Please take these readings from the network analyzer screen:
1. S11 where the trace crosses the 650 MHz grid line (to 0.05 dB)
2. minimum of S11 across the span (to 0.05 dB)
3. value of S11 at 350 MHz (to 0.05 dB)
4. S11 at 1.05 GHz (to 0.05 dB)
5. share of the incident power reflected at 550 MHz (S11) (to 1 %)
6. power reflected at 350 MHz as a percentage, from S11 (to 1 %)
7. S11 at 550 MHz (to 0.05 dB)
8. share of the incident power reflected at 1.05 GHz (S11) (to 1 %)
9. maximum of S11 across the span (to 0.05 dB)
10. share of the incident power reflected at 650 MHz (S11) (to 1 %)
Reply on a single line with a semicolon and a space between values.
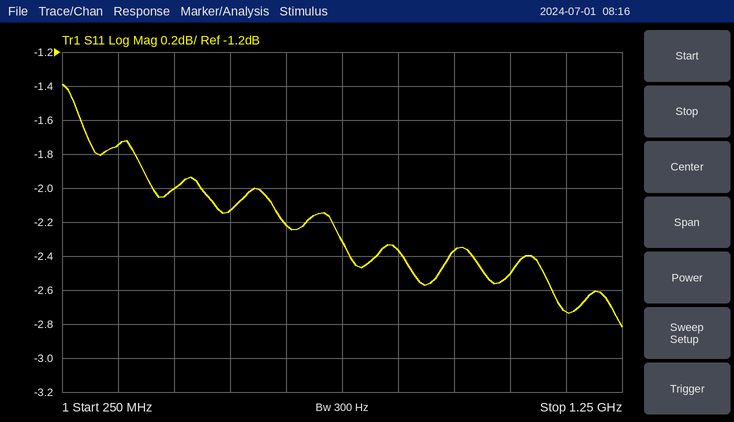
-2.20 dB; -2.80 dB; -1.75 dB; -2.50 dB; 61 %; 67 %; -2.15 dB; 56 %; -1.40 dB; 60 %
